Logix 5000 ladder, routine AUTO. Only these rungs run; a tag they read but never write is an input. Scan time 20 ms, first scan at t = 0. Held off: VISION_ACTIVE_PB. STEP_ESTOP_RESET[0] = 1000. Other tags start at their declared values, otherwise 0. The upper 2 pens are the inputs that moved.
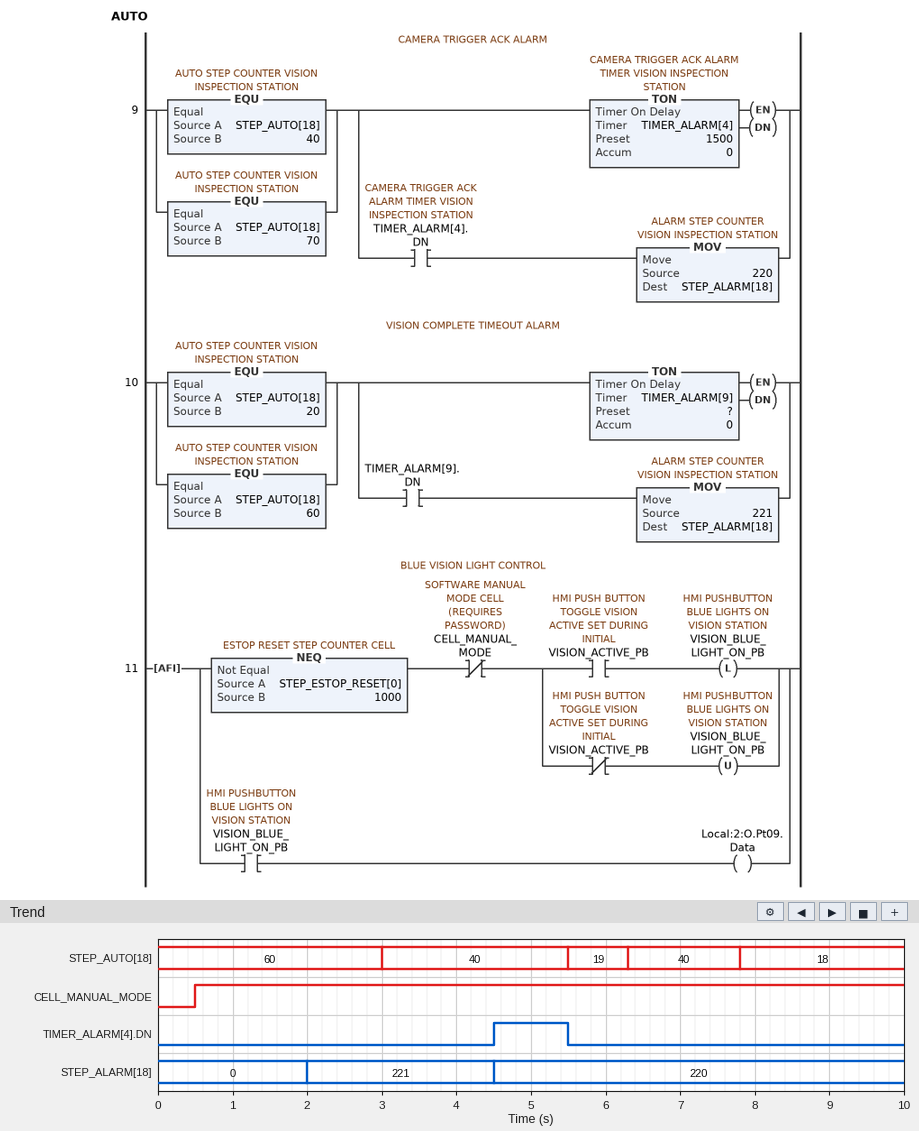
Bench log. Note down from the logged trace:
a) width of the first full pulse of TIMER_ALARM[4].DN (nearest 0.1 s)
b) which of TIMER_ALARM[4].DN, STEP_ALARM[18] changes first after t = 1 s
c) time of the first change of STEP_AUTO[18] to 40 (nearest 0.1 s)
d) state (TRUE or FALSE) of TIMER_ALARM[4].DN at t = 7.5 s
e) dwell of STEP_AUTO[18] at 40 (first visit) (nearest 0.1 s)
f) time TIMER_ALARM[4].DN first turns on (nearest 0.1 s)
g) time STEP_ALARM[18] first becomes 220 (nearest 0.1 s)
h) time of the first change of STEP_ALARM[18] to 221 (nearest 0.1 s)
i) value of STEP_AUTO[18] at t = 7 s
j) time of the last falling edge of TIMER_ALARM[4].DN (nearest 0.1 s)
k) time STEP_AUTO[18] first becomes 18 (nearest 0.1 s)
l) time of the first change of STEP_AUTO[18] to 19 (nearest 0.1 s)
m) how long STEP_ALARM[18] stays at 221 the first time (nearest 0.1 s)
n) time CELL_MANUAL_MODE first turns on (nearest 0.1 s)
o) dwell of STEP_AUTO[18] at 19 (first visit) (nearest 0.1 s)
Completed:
1.0 s
STEP_ALARM[18]
3.0 s
FALSE
2.5 s
4.5 s
4.5 s
2.0 s
40
5.5 s
7.8 s
5.5 s
2.5 s
0.5 s
0.8 s
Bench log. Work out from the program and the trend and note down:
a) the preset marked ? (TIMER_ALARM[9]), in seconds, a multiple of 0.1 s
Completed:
2.0 s
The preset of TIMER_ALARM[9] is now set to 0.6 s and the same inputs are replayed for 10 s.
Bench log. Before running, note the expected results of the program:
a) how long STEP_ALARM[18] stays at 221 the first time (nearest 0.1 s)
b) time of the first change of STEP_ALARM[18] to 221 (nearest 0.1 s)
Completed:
3.9 s
0.6 s
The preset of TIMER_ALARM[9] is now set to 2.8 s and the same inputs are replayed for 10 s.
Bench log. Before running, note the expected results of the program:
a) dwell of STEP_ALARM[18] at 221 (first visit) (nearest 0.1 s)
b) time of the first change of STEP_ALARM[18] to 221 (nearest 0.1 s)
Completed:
1.7 s
2.8 s
